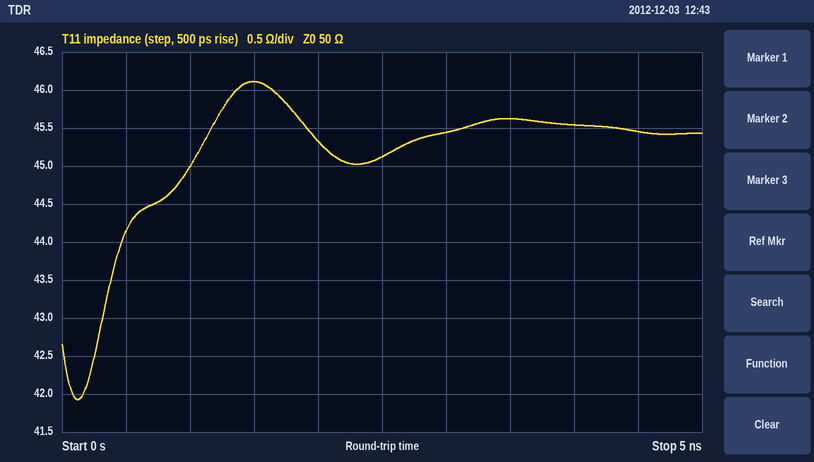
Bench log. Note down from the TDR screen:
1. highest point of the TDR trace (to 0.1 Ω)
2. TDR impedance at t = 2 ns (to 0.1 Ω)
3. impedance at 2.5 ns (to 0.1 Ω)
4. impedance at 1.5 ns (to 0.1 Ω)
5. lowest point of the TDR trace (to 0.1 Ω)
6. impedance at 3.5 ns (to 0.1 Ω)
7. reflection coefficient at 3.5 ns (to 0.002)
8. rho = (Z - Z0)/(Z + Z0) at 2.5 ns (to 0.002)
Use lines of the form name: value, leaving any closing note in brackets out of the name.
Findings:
highest point of the TDR trace: 46.1 Ω
TDR impedance at t = 2 ns: 45.3 Ω
impedance at 2.5 ns: 45.1 Ω
impedance at 1.5 ns: 46.1 Ω
lowest point of the TDR trace: 41.9 Ω
impedance at 3.5 ns: 45.6 Ω
reflection coefficient at 3.5 ns: -0.046
rho = (Z - Z0)/(Z + Z0) at 2.5 ns: -0.052
